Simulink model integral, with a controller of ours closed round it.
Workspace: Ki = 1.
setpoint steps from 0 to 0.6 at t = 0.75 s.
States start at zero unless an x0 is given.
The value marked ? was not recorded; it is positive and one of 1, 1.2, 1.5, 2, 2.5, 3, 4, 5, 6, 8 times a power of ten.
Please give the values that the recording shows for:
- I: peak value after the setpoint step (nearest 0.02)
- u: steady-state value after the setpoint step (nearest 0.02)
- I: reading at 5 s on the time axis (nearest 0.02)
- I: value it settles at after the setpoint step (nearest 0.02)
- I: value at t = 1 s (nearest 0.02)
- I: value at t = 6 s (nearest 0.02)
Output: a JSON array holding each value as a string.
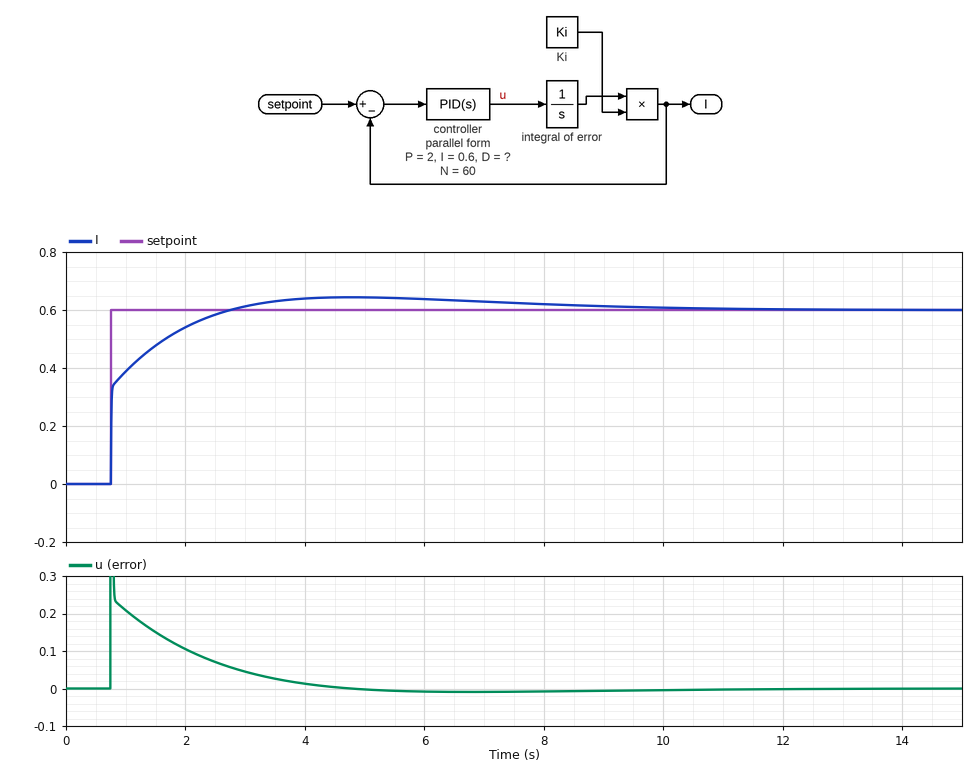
["0.64", "0.00", "0.64", "0.60", "0.38", "0.64"]
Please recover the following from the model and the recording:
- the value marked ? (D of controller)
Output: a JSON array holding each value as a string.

["1.2"]
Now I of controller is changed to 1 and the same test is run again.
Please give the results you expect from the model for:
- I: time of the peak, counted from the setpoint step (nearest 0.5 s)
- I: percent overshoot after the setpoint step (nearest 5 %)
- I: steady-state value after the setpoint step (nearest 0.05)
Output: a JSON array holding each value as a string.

["3.5 s", "10 %", "0.60"]
